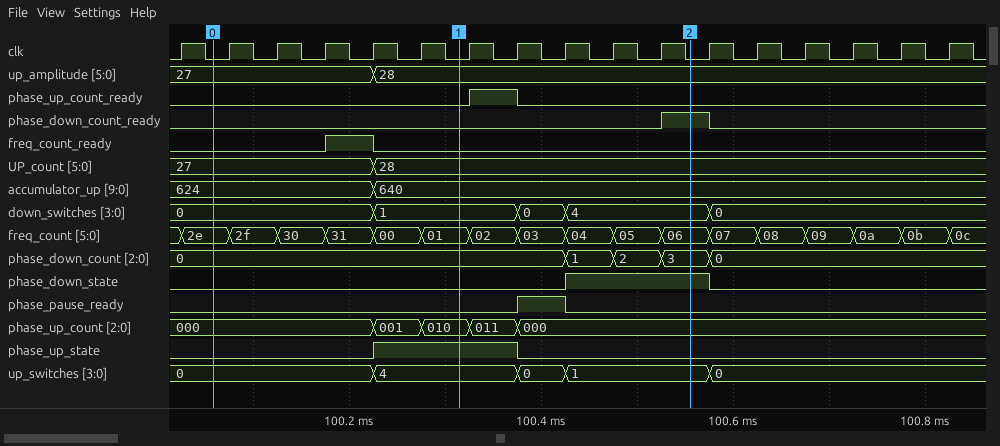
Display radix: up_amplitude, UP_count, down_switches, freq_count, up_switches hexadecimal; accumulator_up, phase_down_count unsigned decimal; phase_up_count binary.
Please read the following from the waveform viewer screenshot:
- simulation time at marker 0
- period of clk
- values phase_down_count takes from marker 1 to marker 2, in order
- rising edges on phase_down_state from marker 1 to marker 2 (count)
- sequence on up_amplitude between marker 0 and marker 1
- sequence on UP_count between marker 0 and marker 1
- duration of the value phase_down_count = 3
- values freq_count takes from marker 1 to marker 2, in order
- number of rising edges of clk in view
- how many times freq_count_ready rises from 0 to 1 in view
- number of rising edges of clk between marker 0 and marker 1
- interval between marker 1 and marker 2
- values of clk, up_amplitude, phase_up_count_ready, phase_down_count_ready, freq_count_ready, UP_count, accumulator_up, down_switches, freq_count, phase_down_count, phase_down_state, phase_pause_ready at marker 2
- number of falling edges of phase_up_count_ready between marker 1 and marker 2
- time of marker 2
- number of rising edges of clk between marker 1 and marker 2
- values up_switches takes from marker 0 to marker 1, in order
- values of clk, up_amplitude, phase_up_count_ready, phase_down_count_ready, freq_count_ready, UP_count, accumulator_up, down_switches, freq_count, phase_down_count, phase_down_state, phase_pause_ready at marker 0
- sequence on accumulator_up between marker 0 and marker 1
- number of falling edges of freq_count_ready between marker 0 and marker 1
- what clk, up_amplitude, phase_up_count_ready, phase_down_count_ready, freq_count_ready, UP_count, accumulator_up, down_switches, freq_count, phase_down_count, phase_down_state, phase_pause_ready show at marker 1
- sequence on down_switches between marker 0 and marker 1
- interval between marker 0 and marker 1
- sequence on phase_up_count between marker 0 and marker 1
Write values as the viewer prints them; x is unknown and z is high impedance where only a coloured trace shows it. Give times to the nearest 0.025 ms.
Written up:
100.05 ms
0.05 ms
0, 1, 2, 3
1
27, 28
27, 28
0.05 ms
01, 02, 03, 04, 05, 06
17
1
5
0.25 ms
clk=0, up_amplitude=28, phase_up_count_ready=0, phase_down_count_ready=1, freq_count_ready=0, UP_count=28, accumulator_up=640, down_switches=4, freq_count=06, phase_down_count=3, phase_down_state=1, phase_pause_ready=0
1
100.55 ms
5
0, 4
clk=0, up_amplitude=27, phase_up_count_ready=0, phase_down_count_ready=0, freq_count_ready=0, UP_count=27, accumulator_up=624, down_switches=0, freq_count=2e, phase_down_count=0, phase_down_state=0, phase_pause_ready=0
624, 640
1
clk=0, up_amplitude=28, phase_up_count_ready=0, phase_down_count_ready=0, freq_count_ready=0, UP_count=28, accumulator_up=640, down_switches=1, freq_count=01, phase_down_count=0, phase_down_state=0, phase_pause_ready=0
0, 1
0.25 ms
000, 001, 010
